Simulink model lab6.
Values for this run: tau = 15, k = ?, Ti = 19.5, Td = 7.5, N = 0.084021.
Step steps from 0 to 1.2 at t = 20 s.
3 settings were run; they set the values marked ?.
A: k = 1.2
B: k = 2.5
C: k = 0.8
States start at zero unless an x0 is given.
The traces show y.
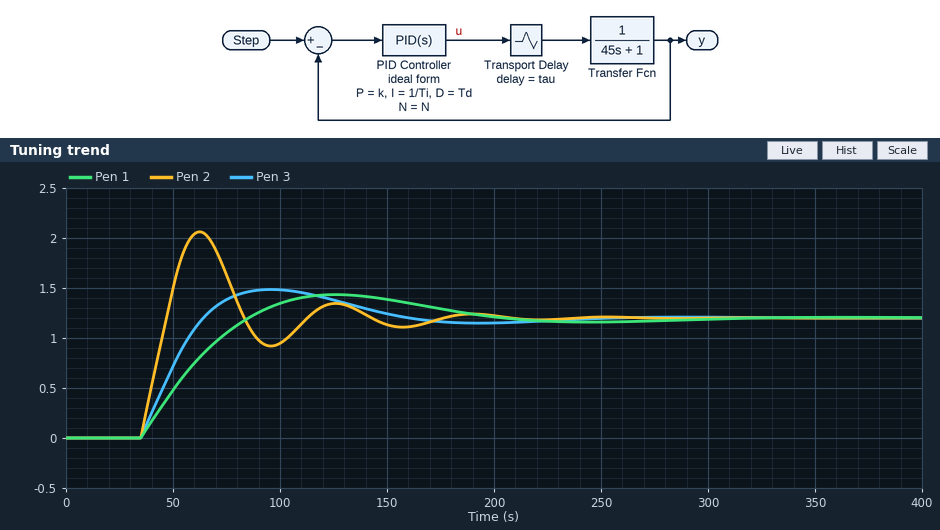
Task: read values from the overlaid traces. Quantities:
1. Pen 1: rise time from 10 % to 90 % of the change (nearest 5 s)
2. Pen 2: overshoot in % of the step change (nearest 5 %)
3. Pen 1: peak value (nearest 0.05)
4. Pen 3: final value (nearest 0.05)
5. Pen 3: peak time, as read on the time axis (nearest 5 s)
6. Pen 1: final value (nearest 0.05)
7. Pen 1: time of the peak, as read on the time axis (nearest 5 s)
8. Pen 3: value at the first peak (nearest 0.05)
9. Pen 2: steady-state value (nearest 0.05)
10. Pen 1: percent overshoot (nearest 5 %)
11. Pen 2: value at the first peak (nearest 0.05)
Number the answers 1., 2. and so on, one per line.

1. 40 s
2. 70 %
3. 1.45
4. 1.20
5. 95 s
6. 1.20
7. 125 s
8. 1.50
9. 1.20
10. 20 %
11. 2.05
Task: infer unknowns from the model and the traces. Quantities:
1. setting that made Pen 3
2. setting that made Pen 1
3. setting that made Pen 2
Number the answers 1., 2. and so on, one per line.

1. A
2. C
3. B
